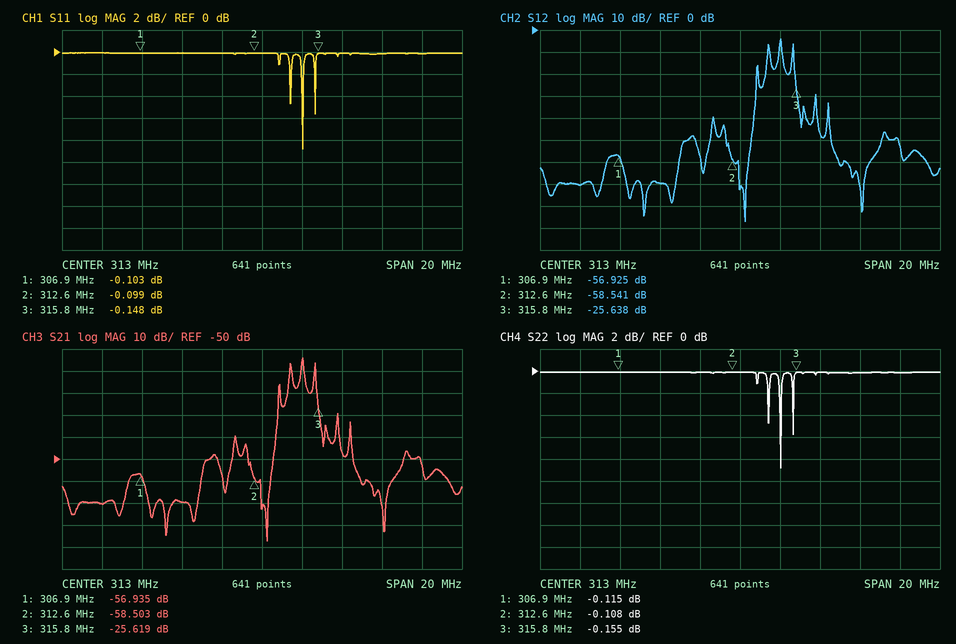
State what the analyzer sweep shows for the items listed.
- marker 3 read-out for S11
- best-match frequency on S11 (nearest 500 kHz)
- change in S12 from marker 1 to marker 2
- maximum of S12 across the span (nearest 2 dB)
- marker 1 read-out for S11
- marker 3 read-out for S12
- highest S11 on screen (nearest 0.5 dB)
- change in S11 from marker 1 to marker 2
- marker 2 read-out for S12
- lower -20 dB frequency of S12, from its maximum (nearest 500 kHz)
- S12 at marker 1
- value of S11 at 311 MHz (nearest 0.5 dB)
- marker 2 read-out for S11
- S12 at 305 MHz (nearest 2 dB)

-0.148 dB
315.0 MHz
-1.616 dB
-4 dB
-0.103 dB
-25.638 dB
0.0 dB
0.004 dB
-58.541 dB
314.0 MHz
-56.925 dB
0.0 dB
-0.099 dB
-70 dB
